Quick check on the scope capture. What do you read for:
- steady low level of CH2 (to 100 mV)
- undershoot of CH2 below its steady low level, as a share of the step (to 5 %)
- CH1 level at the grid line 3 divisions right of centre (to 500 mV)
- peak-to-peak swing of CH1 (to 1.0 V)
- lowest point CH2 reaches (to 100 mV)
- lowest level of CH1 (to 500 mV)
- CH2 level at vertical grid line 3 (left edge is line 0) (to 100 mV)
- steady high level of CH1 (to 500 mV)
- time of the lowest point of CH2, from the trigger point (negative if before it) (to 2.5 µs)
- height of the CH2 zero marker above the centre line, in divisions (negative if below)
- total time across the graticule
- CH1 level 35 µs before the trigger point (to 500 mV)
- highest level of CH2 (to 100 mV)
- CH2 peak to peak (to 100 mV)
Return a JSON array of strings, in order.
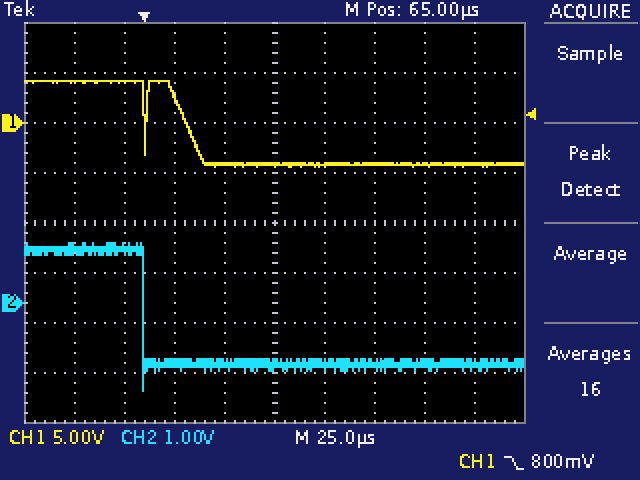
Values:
["-1.2 V", "25 %", "-4.0 V", "9.0 V", "-1.8 V", "-4.5 V", "-1.2 V", "4.0 V", "0.0 µs", "-1.6 div", "250 µs", "4.0 V", "1.2 V", "3.0 V"]
